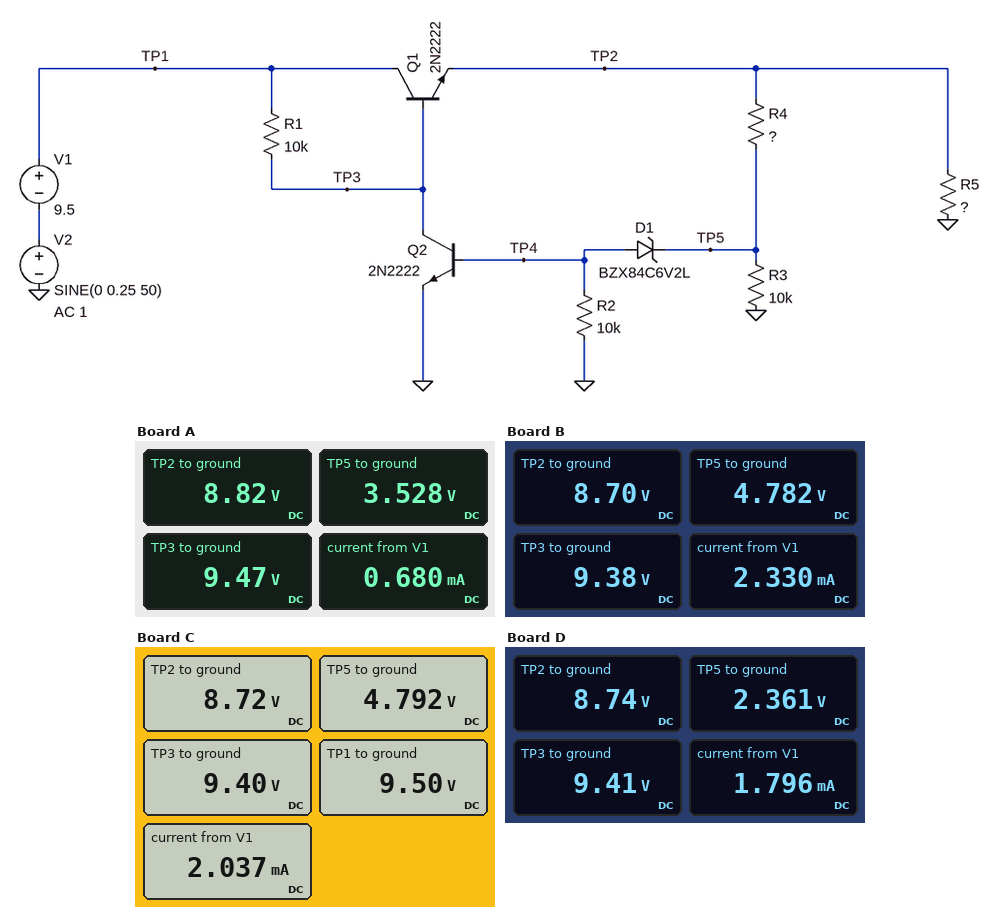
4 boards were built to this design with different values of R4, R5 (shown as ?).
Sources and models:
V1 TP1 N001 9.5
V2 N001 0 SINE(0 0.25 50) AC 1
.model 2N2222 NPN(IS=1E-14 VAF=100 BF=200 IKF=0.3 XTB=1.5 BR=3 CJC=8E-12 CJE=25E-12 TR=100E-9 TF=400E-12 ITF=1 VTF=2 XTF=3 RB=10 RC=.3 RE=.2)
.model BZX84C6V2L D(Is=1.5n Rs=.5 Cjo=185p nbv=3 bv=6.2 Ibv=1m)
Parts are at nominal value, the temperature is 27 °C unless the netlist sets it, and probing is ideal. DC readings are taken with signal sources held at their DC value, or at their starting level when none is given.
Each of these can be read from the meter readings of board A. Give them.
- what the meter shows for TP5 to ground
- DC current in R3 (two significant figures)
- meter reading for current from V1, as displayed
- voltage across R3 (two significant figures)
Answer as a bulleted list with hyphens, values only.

- 3.528 V
- 350 µA
- 0.680 mA
- 3.5 V
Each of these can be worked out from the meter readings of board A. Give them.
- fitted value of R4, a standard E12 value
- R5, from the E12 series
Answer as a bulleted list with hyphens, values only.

- 15 kΩ
- 27 kΩ
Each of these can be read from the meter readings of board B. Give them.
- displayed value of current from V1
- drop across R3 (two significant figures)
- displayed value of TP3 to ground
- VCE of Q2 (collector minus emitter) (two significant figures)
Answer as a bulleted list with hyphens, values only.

- 2.330 mA
- 4.8 V
- 9.38 V
- 9.4 V
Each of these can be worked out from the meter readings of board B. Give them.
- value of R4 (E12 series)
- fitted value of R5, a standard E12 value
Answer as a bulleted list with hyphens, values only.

- 8.2 kΩ
- 4.7 kΩ
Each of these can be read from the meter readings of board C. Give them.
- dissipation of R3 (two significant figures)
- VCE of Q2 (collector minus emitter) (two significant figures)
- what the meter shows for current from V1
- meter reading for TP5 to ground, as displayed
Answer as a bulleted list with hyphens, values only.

- 2.3 mW
- 9.4 V
- 2.037 mA
- 4.792 V
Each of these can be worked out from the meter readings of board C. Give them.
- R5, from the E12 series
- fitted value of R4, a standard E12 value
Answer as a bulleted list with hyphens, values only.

- 5.6 kΩ
- 8.2 kΩ
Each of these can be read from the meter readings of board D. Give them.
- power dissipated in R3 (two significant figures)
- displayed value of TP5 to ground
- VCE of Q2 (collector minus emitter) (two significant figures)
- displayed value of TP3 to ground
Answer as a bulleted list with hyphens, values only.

- 560 µW
- 2.361 V
- 9.4 V
- 9.41 V
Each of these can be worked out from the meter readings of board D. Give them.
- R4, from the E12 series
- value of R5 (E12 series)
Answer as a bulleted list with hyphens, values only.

- 27 kΩ
- 5.6 kΩ
